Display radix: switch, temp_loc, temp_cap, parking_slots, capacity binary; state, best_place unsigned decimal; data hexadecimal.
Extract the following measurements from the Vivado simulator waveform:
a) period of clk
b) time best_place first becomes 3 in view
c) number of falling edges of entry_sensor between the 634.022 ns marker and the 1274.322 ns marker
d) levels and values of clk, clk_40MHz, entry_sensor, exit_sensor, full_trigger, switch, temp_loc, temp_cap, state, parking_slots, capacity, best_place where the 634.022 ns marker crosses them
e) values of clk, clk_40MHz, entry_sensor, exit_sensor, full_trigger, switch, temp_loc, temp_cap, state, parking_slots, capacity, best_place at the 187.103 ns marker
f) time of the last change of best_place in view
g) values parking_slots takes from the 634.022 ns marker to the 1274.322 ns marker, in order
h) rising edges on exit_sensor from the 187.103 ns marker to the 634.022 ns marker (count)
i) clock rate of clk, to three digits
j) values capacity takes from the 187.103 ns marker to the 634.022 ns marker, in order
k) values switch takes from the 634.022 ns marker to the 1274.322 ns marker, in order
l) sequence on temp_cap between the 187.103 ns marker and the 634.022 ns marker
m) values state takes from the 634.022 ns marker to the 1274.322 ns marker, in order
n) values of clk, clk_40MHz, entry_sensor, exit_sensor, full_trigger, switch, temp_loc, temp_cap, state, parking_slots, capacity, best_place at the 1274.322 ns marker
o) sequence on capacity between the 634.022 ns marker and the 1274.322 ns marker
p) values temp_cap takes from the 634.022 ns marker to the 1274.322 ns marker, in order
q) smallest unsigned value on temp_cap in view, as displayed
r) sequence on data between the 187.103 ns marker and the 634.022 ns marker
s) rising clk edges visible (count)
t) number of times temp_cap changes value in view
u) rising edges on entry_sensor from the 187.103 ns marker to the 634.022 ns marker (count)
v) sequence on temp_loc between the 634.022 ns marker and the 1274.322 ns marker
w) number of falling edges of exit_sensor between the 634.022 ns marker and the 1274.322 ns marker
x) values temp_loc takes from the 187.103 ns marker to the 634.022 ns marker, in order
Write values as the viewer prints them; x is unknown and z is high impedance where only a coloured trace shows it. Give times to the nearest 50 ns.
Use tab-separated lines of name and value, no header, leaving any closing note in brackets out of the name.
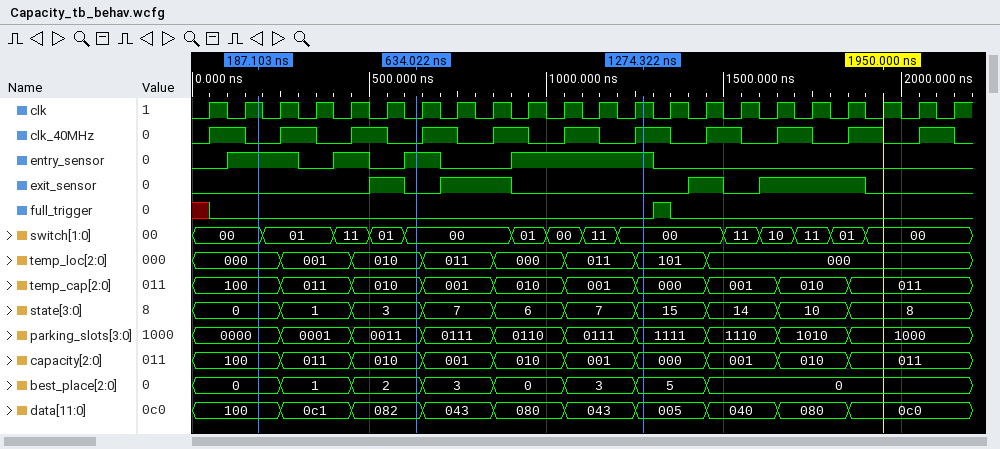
period of clk	100 ns
time best_place first becomes 3 in view	650 ns
number of falling edges of entry_sensor between the 634.022 ns marker and the 1274.322 ns marker	1
levels and values of clk, clk_40MHz, entry_sensor, exit_sensor, full_trigger, switch, temp_loc, temp_cap, state, parking_slots, capacity, best_place where the 634.022 ns marker crosses them	clk=0, clk_40MHz=0, entry_sensor=1, exit_sensor=0, full_trigger=0, switch=00, temp_loc=010, temp_cap=010, state=3, parking_slots=0011, capacity=010, best_place=2
values of clk, clk_40MHz, entry_sensor, exit_sensor, full_trigger, switch, temp_loc, temp_cap, state, parking_slots, capacity, best_place at the 187.103 ns marker	clk=1, clk_40MHz=0, entry_sensor=1, exit_sensor=0, full_trigger=0, switch=00, temp_loc=000, temp_cap=100, state=0, parking_slots=0000, capacity=100, best_place=0
time of the last change of best_place in view	1450 ns
values parking_slots takes from the 634.022 ns marker to the 1274.322 ns marker, in order	0011, 0111, 0110, 0111, 1111
rising edges on exit_sensor from the 187.103 ns marker to the 634.022 ns marker	1
clock rate of clk, to three digits	10.0 MHz
values capacity takes from the 187.103 ns marker to the 634.022 ns marker, in order	100, 011, 010
values switch takes from the 634.022 ns marker to the 1274.322 ns marker, in order	00, 01, 00, 11, 00
sequence on temp_cap between the 187.103 ns marker and the 634.022 ns marker	100, 011, 010
values state takes from the 634.022 ns marker to the 1274.322 ns marker, in order	3, 7, 6, 7, 15
values of clk, clk_40MHz, entry_sensor, exit_sensor, full_trigger, switch, temp_loc, temp_cap, state, parking_slots, capacity, best_place at the 1274.322 ns marker	clk=1, clk_40MHz=1, entry_sensor=1, exit_sensor=0, full_trigger=0, switch=00, temp_loc=101, temp_cap=000, state=15, parking_slots=1111, capacity=000, best_place=5
sequence on capacity between the 634.022 ns marker and the 1274.322 ns marker	010, 001, 010, 001, 000
values temp_cap takes from the 634.022 ns marker to the 1274.322 ns marker, in order	010, 001, 010, 001, 000
smallest unsigned value on temp_cap in view, as displayed	000
sequence on data between the 187.103 ns marker and the 634.022 ns marker	100, 0c1, 082
rising clk edges visible	22
number of times temp_cap changes value in view	9
rising edges on entry_sensor from the 187.103 ns marker to the 634.022 ns marker	2
sequence on temp_loc between the 634.022 ns marker and the 1274.322 ns marker	010, 011, 000, 011, 101
number of falling edges of exit_sensor between the 634.022 ns marker and the 1274.322 ns marker	1
values temp_loc takes from the 187.103 ns marker to the 634.022 ns marker, in order	000, 001, 010
